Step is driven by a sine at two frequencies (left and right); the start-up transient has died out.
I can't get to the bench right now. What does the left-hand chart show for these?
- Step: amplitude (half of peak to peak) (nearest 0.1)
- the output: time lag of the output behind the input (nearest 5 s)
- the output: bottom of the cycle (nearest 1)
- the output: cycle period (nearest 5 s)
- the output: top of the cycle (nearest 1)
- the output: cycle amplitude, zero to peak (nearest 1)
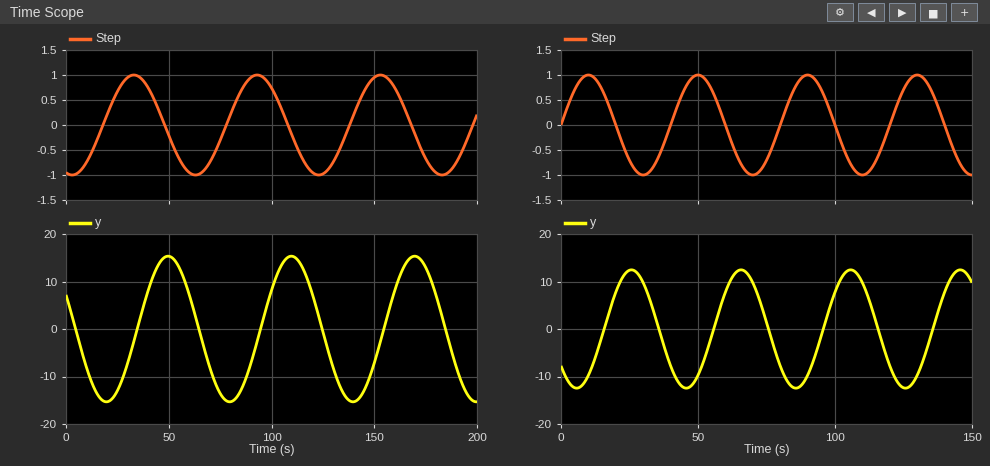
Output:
1.0
15 s
-15
60 s
15
15
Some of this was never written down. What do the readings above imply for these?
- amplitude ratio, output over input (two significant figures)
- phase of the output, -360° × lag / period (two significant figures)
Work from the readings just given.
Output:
15
-90°
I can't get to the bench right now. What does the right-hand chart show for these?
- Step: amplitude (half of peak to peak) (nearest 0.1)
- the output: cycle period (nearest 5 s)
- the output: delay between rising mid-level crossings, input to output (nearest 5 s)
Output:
1.0
40 s
15 s
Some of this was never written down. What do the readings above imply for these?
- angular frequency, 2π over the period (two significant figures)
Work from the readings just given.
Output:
0.16 rad/s
